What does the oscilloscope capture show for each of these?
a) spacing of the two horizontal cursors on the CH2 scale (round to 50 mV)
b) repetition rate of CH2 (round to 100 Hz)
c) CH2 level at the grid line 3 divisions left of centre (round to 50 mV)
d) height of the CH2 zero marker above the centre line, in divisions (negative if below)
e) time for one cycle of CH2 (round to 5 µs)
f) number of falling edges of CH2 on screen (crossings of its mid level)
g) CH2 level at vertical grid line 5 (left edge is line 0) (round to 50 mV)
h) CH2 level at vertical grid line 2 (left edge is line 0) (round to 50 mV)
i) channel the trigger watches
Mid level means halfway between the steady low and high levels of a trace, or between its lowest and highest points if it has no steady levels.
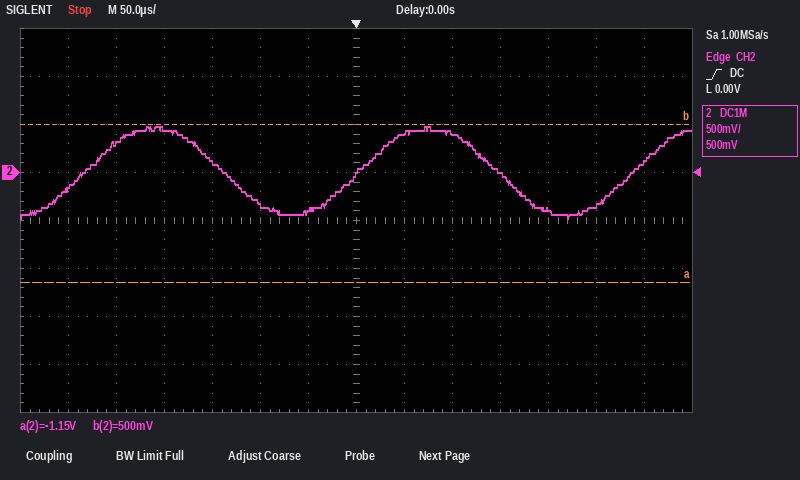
1.65 V
3.5 kHz
100 mV
+1.0 div
285 µs
2
-350 mV
300 mV
CH2
